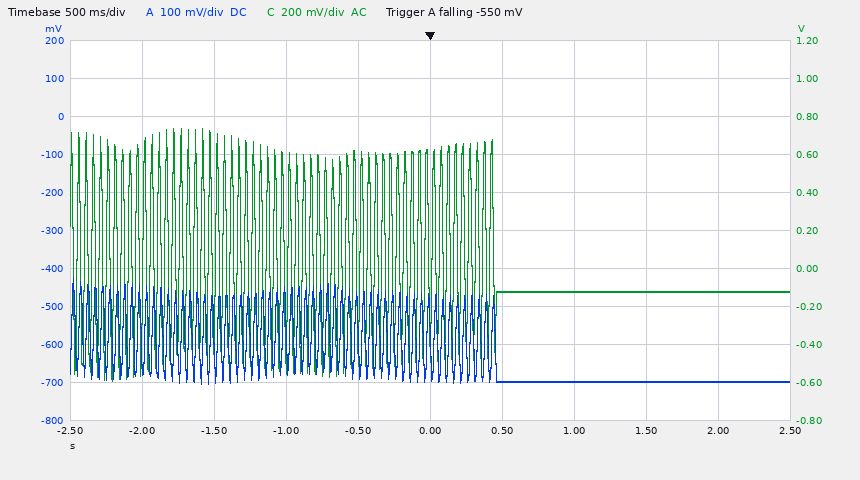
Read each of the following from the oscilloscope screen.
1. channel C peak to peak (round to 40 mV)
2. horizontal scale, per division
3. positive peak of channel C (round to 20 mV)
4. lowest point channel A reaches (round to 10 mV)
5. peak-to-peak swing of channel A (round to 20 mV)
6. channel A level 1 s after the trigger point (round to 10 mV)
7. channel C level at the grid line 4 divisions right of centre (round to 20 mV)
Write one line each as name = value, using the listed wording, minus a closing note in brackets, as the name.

channel C peak to peak = 1.32 V
horizontal scale, per division = 500 ms
positive peak of channel C = 740 mV
lowest point channel A reaches = -700 mV
peak-to-peak swing of channel A = 280 mV
channel A level 1 s after the trigger point = -700 mV
channel C level at the grid line 4 divisions right of centre = -120 mV
